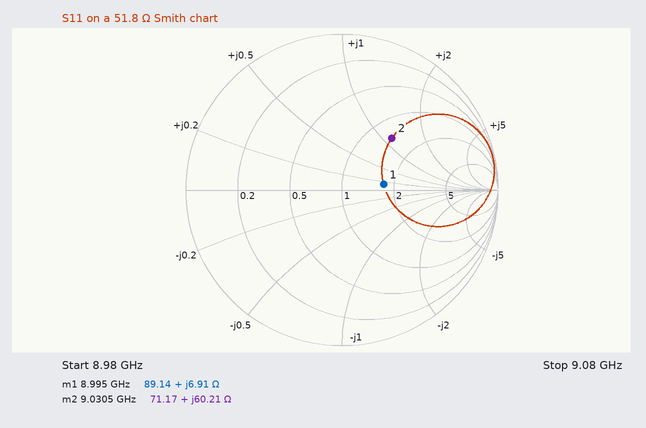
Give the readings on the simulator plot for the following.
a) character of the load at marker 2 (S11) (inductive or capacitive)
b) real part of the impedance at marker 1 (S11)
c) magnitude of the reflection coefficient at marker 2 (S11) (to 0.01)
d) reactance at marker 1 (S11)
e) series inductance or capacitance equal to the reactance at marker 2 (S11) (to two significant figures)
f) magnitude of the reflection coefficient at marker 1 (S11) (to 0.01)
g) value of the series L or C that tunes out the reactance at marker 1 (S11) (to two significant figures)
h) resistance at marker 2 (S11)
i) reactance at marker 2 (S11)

inductive
89.14 Ω
0.46
+6.91 Ω
1.1 nH
0.27
2.6 pF
71.17 Ω
+60.21 Ω
